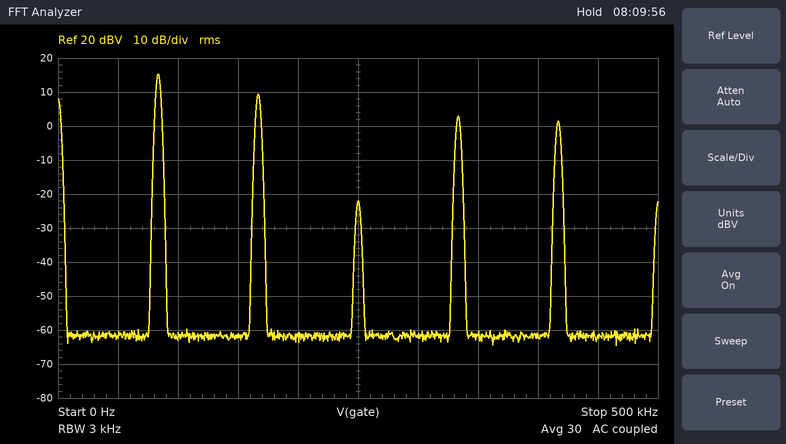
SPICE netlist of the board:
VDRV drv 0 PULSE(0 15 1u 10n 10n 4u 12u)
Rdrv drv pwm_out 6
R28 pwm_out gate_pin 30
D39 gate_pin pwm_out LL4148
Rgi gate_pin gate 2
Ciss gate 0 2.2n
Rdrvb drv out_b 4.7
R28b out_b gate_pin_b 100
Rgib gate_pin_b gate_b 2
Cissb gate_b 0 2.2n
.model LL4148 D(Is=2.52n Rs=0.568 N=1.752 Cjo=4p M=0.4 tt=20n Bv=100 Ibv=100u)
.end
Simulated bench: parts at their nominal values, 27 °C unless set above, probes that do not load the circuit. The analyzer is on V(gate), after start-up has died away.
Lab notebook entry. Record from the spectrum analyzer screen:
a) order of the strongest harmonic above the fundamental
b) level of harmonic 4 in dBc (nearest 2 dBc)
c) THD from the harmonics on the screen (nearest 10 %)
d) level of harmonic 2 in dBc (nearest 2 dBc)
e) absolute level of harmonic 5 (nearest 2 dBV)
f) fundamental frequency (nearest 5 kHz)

2
-12 dBc
60 %
-6 dBc
2 dBV
85 kHz
